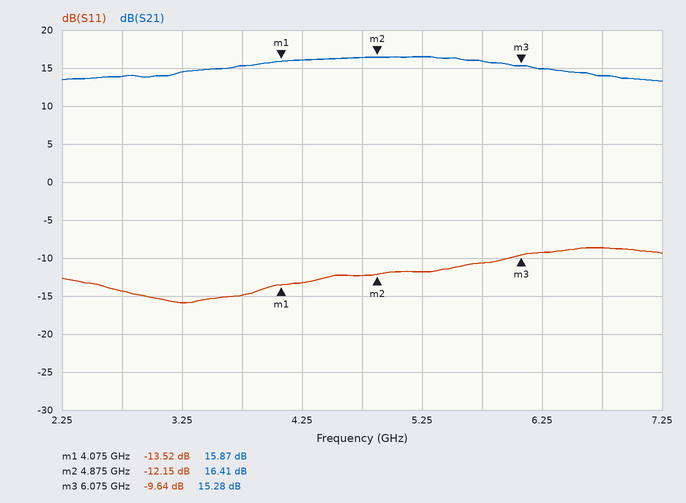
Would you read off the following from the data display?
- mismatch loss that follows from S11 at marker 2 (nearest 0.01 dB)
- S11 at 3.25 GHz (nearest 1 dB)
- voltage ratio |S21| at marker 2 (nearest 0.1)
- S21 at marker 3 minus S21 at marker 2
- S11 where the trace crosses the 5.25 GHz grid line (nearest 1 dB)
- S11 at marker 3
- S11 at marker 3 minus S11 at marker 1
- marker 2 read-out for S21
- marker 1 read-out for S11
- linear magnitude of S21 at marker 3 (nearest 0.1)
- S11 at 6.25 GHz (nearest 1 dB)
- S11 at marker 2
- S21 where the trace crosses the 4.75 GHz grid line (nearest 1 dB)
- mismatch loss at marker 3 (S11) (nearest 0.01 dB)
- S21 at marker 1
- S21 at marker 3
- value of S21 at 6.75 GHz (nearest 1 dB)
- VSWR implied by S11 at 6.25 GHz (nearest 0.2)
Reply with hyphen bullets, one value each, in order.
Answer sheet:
- 0.27 dB
- -16 dB
- 6.6
- -1.13 dB
- -12 dB
- -9.64 dB
- 3.88 dB
- 16.41 dB
- -13.52 dB
- 5.8
- -9 dB
- -12.15 dB
- 16 dB
- 0.50 dB
- 15.87 dB
- 15.28 dB
- 14 dB
- 2.0
